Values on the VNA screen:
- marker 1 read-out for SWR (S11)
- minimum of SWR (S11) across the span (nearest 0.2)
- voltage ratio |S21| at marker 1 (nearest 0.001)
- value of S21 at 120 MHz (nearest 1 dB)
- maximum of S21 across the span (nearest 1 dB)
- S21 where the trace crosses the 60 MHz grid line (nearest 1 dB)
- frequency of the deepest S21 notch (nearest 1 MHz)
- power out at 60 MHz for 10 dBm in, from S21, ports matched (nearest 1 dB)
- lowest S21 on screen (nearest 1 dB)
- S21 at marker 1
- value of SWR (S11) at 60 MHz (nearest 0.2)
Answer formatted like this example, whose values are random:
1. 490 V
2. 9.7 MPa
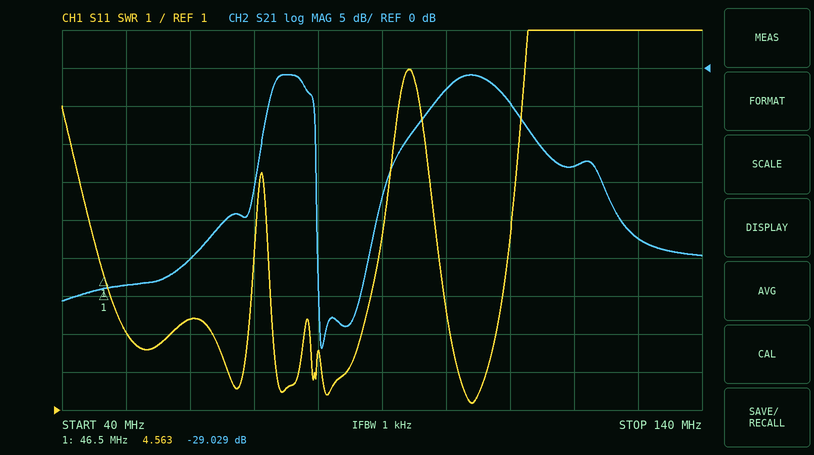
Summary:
1. 4.563
2. 1.2
3. 0.035
4. -13 dB
5. -1 dB
6. -25 dB
7. 81 MHz
8. -15 dBm
9. -37 dB
10. -29.029 dB
11. 3.4
